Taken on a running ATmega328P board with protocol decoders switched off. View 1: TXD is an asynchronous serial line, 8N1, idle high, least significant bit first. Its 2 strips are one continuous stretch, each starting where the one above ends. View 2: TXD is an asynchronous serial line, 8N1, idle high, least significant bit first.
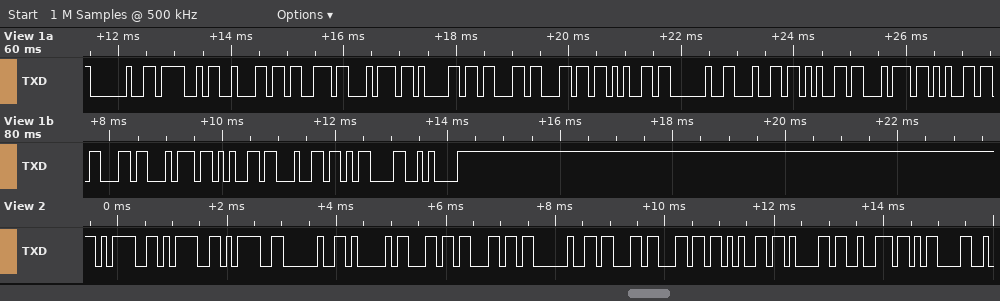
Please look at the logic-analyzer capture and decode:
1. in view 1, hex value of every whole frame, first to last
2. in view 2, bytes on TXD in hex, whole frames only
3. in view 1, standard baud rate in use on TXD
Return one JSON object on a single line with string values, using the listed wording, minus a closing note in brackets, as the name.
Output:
{"in view 1, hex value of every whole frame, first to last": "20 4F 62 73 74 61 63 6C 65 20 64 65 74 65 63 74 65 64 0D 0A", "in view 2, bytes on TXD in hex, whole frames only": "3D 3D 3D 20 41 6C 6C 20 63 6C 65 61 72 0D", "in view 1, standard baud rate in use on TXD": "9600 baud"}
